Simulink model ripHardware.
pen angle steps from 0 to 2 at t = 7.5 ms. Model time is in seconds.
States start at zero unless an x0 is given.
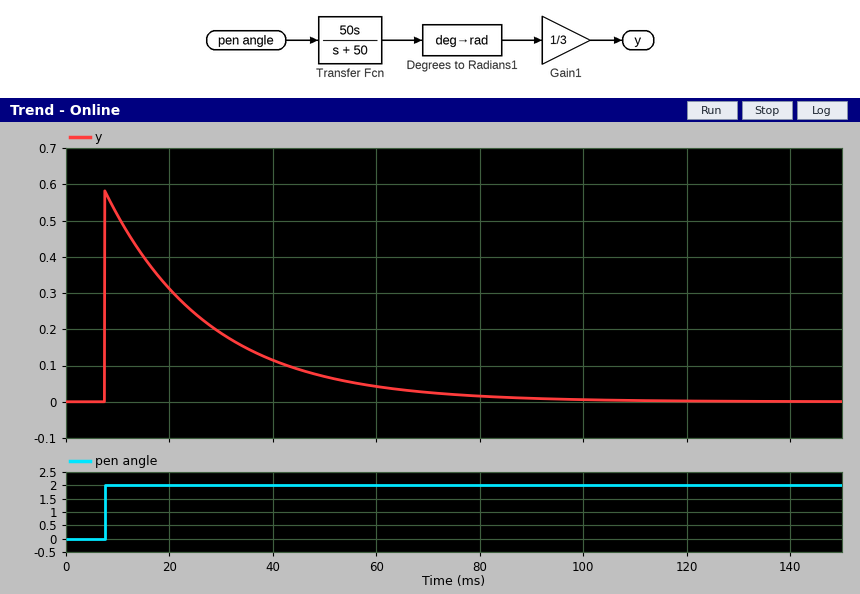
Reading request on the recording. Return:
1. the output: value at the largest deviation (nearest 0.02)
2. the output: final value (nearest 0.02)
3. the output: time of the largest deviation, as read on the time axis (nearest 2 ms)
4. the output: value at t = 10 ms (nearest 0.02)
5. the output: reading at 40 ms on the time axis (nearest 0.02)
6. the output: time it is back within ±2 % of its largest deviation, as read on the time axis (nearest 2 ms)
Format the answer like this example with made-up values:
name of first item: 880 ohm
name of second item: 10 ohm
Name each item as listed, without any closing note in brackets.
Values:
the output: value at the largest deviation: 0.58
the output: final value: 0.00
the output: time of the largest deviation, as read on the time axis: 8 ms
the output: value at t = 10 ms: 0.52
the output: reading at 40 ms on the time axis: 0.12
the output: time it is back within ±2 % of its largest deviation, as read on the time axis: 86 ms
